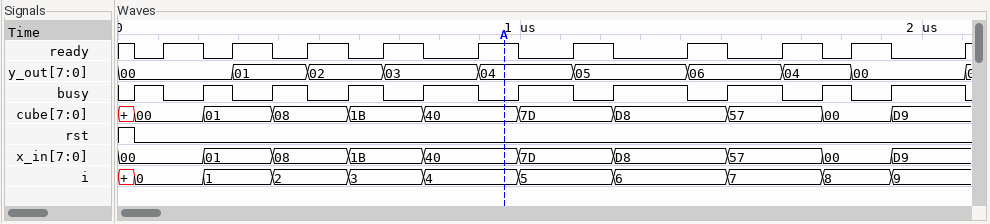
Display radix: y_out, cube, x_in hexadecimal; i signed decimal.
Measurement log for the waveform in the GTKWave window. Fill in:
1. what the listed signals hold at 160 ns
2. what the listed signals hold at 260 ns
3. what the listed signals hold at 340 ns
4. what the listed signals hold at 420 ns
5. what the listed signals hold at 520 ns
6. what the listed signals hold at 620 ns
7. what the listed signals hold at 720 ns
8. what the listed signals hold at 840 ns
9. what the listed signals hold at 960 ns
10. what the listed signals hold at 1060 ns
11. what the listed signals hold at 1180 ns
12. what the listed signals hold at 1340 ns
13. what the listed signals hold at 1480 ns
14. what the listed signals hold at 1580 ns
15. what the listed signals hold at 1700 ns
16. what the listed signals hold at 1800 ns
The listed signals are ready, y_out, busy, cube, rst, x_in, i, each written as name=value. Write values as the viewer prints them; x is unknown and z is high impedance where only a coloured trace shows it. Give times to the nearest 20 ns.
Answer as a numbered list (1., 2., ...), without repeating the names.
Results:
1. ready=1, y_out=00, busy=0, cube=00, rst=0, x_in=00, i=0
2. ready=0, y_out=00, busy=1, cube=01, rst=0, x_in=01, i=1
3. ready=1, y_out=01, busy=0, cube=01, rst=0, x_in=01, i=1
4. ready=0, y_out=01, busy=1, cube=08, rst=0, x_in=08, i=2
5. ready=1, y_out=02, busy=0, cube=08, rst=0, x_in=08, i=2
6. ready=0, y_out=02, busy=1, cube=1B, rst=0, x_in=1B, i=3
7. ready=1, y_out=03, busy=0, cube=1B, rst=0, x_in=1B, i=3
8. ready=0, y_out=03, busy=1, cube=40, rst=0, x_in=40, i=4
9. ready=1, y_out=04, busy=0, cube=40, rst=0, x_in=40, i=4
10. ready=0, y_out=04, busy=1, cube=7D, rst=0, x_in=7D, i=5
11. ready=1, y_out=05, busy=0, cube=7D, rst=0, x_in=7D, i=5
12. ready=0, y_out=05, busy=1, cube=D8, rst=0, x_in=D8, i=6
13. ready=1, y_out=06, busy=0, cube=D8, rst=0, x_in=D8, i=6
14. ready=0, y_out=06, busy=1, cube=57, rst=0, x_in=57, i=7
15. ready=1, y_out=04, busy=0, cube=57, rst=0, x_in=57, i=7
16. ready=0, y_out=04, busy=1, cube=00, rst=0, x_in=00, i=8
